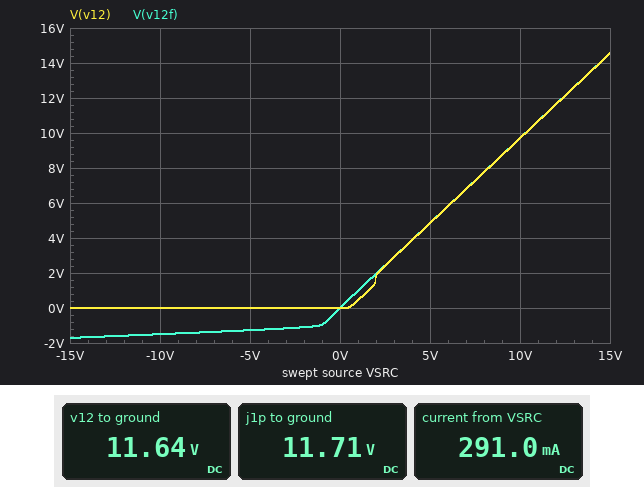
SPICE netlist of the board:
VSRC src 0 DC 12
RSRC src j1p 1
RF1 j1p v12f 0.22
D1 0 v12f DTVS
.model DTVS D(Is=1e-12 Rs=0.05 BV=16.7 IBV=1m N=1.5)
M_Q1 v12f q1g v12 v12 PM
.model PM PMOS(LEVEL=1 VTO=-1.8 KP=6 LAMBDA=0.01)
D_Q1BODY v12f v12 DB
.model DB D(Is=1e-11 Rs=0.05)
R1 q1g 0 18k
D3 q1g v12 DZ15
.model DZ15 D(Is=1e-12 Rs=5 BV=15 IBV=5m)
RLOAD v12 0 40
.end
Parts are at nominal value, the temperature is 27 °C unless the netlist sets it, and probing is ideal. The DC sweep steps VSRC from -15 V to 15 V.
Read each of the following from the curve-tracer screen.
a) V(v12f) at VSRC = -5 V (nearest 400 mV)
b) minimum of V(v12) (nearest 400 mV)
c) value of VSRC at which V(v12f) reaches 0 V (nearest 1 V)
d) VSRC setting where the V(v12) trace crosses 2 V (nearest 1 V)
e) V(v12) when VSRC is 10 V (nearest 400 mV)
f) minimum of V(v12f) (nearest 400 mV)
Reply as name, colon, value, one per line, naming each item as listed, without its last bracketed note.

V(v12f) at VSRC = -5 V: -1.2 V
minimum of V(v12): 0 V
value of VSRC at which V(v12f) reaches 0 V: 0 V
VSRC setting where the V(v12) trace crosses 2 V: 2 V
V(v12) when VSRC is 10 V: 9.6 V
minimum of V(v12f): -1.6 V
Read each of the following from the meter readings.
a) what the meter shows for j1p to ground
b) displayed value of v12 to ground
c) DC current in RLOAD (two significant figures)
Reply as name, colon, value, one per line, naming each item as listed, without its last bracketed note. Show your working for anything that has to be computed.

what the meter shows for j1p to ground: 11.71 V
displayed value of v12 to ground: 11.64 V
DC current in RLOAD: (11.64 V) / 40 Ω = 290 mA
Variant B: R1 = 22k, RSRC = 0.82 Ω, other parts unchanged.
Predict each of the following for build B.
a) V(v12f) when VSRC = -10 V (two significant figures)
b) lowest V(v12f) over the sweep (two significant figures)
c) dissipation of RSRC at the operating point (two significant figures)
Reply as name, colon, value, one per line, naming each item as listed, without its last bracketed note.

V(v12f) when VSRC = -10 V: -1.6 V
lowest V(v12f) over the sweep: -1.8 V
dissipation of RSRC at the operating point: 70 mW
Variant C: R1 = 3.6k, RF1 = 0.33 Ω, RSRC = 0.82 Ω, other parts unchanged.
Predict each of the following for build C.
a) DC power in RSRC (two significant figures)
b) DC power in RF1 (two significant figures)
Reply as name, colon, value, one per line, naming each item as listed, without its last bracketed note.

DC power in RSRC: 70 mW
DC power in RF1: 28 mW
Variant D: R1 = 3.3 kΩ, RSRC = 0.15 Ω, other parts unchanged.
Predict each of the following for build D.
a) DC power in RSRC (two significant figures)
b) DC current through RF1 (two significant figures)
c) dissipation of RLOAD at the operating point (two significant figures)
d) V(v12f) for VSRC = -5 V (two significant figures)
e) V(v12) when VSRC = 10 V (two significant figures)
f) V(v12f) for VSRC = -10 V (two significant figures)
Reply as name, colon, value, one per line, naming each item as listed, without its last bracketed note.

DC power in RSRC: 13 mW
DC current through RF1: 300 mA
dissipation of RLOAD at the operating point: 3.5 W
V(v12f) for VSRC = -5 V: -1.6 V
V(v12) when VSRC = 10 V: 9.9 V
V(v12f) for VSRC = -10 V: -2.2 V
